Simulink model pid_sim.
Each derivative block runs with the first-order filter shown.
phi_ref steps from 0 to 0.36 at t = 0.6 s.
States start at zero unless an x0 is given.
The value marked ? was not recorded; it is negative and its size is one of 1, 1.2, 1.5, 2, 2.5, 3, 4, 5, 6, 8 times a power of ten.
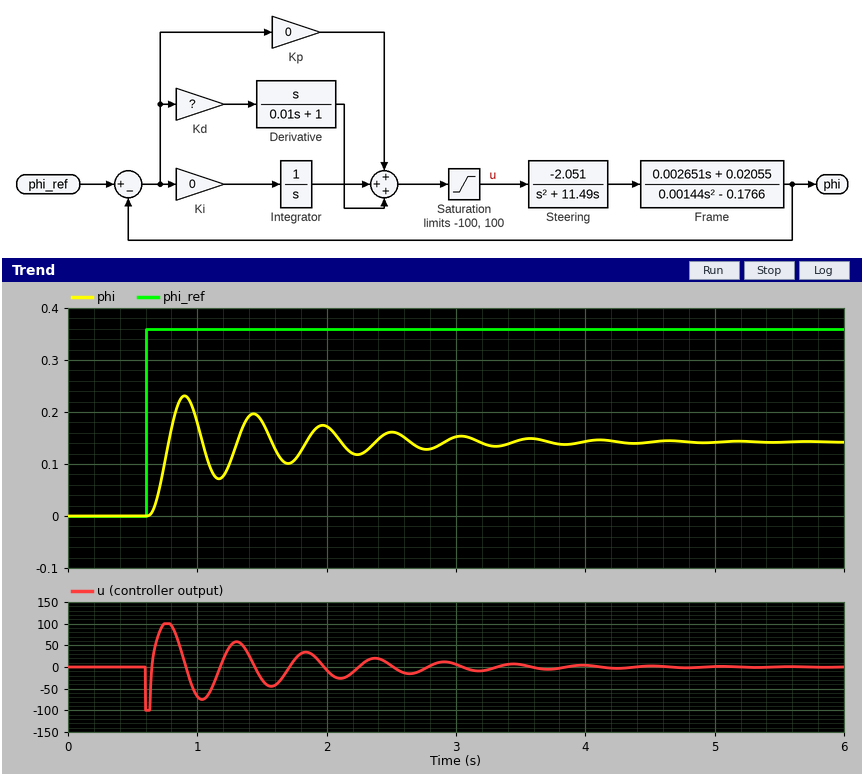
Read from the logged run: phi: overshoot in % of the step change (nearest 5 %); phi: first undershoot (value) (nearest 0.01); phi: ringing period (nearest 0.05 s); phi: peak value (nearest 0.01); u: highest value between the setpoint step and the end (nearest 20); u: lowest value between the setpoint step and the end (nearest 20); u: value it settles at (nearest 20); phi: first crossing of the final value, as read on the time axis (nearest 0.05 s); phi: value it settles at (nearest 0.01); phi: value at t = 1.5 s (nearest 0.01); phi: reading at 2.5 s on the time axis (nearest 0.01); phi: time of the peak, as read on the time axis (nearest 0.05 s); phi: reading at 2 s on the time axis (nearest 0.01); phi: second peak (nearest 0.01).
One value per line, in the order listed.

60 %
0.07
0.55 s
0.23
100
-100
0
0.80 s
0.14
0.18
0.16
0.90 s
0.17
0.20
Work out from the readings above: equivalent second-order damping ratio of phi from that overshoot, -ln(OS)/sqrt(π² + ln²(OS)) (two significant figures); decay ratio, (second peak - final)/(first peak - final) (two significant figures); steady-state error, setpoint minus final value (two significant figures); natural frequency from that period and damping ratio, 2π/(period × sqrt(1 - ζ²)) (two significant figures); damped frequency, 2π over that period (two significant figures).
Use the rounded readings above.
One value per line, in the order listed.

0.16
0.67
0.22
12 rad/s
11 rad/s
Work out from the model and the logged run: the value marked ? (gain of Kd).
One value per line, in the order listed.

-80
